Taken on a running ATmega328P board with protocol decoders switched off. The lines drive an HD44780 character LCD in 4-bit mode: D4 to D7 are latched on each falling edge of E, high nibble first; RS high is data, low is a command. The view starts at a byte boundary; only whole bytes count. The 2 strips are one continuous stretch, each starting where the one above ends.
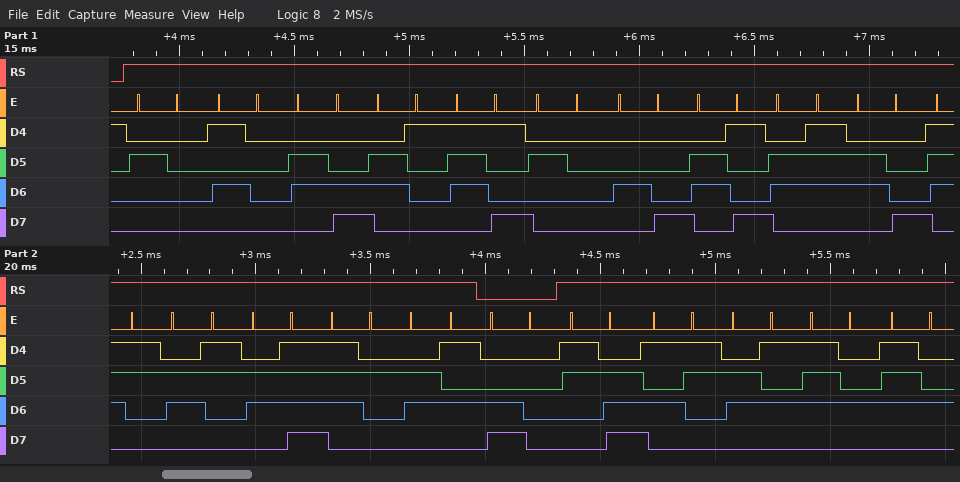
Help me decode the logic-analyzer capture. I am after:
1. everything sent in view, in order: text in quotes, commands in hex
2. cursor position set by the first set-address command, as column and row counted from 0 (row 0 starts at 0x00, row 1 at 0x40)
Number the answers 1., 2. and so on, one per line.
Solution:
1. " Play Highscore" 0xC0 ">Sett"
2. column 0, row 1
